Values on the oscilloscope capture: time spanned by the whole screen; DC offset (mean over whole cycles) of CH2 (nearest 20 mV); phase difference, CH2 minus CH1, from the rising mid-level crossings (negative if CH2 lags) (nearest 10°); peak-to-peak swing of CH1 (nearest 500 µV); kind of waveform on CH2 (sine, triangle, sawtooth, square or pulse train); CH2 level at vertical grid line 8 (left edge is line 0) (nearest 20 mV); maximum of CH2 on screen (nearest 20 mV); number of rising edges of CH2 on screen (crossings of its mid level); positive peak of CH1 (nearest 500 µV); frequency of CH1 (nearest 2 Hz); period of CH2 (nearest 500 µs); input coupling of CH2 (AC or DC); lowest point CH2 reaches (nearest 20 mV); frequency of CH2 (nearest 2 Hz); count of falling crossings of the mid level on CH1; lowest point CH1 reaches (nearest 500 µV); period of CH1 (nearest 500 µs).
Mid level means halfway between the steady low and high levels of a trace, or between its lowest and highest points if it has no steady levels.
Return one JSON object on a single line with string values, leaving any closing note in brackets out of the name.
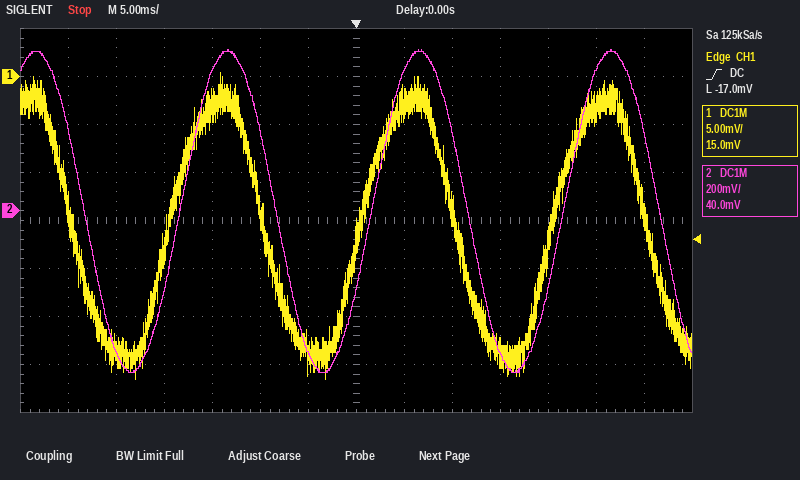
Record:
{"time spanned by the whole screen": "70 ms", "DC offset (mean over whole cycles) of CH2": "0 mV", "phase difference, CH2 minus CH1, from the rising mid-level crossings (negative if CH2 lags)": "-20°", "peak-to-peak swing of CH1": "32.0 mV", "kind of waveform on CH2": "sine", "CH2 level at vertical grid line 8 (left edge is line 0)": "580 mV", "maximum of CH2 on screen": "680 mV", "number of rising edges of CH2 on screen": "3", "positive peak of CH1": "500 µV", "frequency of CH1": "50 Hz", "period of CH2": "20.0 ms", "input coupling of CH2": "DC", "lowest point CH2 reaches": "-680 mV", "frequency of CH2": "50 Hz", "count of falling crossings of the mid level on CH1": "4", "lowest point CH1 reaches": "-31.5 mV", "period of CH1": "20.0 ms"}
